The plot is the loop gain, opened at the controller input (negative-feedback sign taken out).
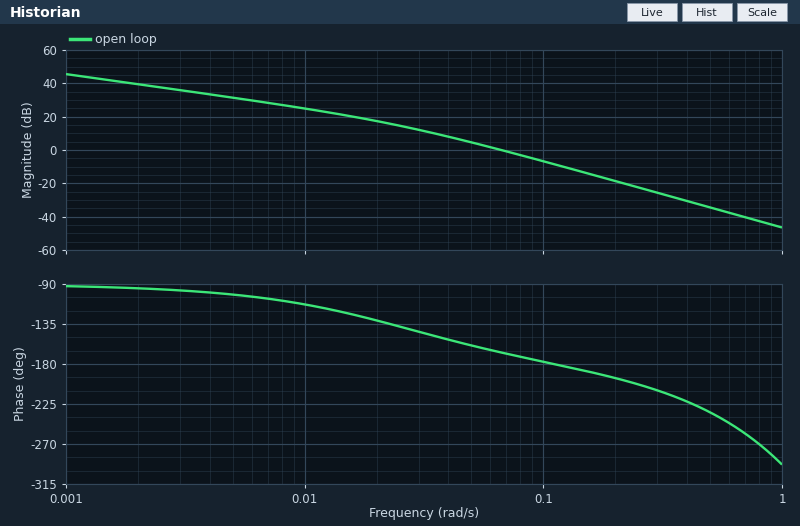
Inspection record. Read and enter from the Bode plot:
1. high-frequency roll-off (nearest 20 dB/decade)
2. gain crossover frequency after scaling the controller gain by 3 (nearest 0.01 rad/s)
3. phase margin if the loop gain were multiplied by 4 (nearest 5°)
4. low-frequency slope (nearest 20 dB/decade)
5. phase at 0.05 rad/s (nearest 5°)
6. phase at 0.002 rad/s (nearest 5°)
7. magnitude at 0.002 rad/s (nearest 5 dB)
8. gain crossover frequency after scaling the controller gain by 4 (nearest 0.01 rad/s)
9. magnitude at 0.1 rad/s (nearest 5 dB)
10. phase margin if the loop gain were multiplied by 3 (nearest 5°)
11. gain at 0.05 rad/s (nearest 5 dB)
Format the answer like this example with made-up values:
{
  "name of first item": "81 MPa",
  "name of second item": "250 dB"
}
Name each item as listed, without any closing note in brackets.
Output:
{
  "high-frequency roll-off": "-40 dB/decade",
  "gain crossover frequency after scaling the controller gain by 3": "0.12 rad/s",
  "phase margin if the loop gain were multiplied by 4": "-5°",
  "low-frequency slope": "-20 dB/decade",
  "phase at 0.05 rad/s": "-160°",
  "phase at 0.002 rad/s": "-95°",
  "magnitude at 0.002 rad/s": "40 dB",
  "gain crossover frequency after scaling the controller gain by 4": "0.14 rad/s",
  "magnitude at 0.1 rad/s": "-5 dB",
  "phase margin if the loop gain were multiplied by 3": "0°",
  "gain at 0.05 rad/s": "5 dB"
}
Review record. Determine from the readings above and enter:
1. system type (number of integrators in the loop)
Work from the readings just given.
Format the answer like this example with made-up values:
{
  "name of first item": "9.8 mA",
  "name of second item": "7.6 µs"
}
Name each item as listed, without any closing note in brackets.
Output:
{
  "system type": "1"
}
